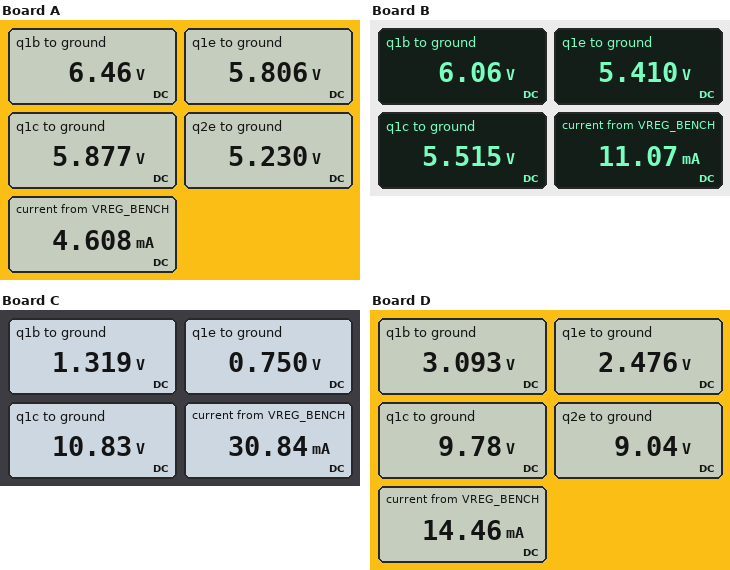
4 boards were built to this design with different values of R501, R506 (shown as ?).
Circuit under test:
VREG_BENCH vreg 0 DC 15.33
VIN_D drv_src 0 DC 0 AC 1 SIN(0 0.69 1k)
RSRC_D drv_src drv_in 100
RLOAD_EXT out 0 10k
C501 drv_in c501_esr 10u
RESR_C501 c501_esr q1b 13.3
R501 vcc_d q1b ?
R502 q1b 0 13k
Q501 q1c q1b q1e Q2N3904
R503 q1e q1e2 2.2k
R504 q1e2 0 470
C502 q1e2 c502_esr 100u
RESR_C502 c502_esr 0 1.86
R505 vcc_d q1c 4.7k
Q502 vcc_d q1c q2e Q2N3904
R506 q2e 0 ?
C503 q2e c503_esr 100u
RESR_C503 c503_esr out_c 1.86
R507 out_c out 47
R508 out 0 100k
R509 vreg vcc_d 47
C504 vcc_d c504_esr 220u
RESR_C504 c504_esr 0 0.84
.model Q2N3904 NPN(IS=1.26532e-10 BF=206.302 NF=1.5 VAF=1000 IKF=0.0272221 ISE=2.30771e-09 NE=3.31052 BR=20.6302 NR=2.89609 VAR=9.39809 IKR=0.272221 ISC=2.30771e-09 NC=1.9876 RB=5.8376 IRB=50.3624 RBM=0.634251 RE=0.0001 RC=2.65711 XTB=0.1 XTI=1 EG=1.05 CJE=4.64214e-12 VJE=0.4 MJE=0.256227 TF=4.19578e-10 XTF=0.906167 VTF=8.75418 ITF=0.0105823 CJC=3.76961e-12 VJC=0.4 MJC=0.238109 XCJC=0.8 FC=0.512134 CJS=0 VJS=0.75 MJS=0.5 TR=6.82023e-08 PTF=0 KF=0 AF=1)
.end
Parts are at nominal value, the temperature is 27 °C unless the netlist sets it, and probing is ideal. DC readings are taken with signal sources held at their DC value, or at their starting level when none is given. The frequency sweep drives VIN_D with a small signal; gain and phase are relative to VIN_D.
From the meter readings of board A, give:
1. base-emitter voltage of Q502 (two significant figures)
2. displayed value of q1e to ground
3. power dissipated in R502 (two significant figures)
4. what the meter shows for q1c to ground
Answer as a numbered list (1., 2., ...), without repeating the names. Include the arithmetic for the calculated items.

1. 5.877 V - 5.23 V = 650 mV
2. 5.806 V
3. (6.46 V)^2 / 13 kΩ = 3.2 mW
4. 5.877 V
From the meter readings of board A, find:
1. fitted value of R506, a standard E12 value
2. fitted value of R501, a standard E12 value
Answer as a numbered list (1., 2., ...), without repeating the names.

1. 2.7 kΩ
2. 12 kΩ
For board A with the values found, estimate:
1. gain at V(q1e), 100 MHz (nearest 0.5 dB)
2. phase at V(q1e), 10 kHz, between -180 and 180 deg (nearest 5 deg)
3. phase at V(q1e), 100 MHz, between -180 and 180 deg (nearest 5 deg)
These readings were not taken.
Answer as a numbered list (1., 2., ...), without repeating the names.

1. -1.0 dB
2. 0 deg
3. -5 deg
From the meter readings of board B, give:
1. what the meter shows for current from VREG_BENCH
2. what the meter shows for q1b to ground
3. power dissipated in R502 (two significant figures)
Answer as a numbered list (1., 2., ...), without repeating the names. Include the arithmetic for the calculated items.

1. 11.07 mA
2. 6.06 V
3. (6.06 V)^2 / 13 kΩ = 2.8 mW
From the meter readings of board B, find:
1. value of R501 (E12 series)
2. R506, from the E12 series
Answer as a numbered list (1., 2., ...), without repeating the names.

1. 15 kΩ
2. 560 Ω
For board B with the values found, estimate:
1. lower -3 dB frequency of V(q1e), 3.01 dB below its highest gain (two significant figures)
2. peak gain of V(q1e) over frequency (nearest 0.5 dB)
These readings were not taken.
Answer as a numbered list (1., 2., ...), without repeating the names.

1. 11 Hz
2. -1.0 dB
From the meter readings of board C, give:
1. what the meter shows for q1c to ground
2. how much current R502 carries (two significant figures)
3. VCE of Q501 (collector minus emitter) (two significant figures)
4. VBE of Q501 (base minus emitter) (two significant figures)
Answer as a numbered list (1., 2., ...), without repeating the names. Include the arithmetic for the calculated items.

1. 10.83 V
2. (1.319 V) / 13 kΩ = 100 µA
3. 10.83 V - 750 mV = 10 V
4. 1.319 V - 750 mV = 570 mV
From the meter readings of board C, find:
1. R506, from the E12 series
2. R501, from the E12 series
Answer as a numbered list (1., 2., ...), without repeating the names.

1. 330 Ω
2. 120 kΩ
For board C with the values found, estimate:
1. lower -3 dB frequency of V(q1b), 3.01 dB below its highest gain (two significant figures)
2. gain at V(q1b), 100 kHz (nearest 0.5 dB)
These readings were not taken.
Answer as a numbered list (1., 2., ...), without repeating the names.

1. 1.4 Hz
2. 0 dB
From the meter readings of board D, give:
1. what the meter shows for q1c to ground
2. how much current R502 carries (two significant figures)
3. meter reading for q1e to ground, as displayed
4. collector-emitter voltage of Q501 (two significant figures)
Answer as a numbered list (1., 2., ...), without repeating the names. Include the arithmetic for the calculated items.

1. 9.78 V
2. (3.093 V) / 13 kΩ = 240 µA
3. 2.476 V
4. 9.78 V - 2.476 V = 7.3 V
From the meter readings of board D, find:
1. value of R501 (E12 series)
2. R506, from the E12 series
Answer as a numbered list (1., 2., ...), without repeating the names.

1. 47 kΩ
2. 680 Ω
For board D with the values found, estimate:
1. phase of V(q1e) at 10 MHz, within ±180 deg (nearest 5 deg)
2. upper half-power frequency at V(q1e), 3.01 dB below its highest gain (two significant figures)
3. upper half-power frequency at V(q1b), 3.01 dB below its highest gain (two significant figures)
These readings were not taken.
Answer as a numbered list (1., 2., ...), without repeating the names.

1. 0 deg
2. 1.2 GHz
3. 1.1 GHz
